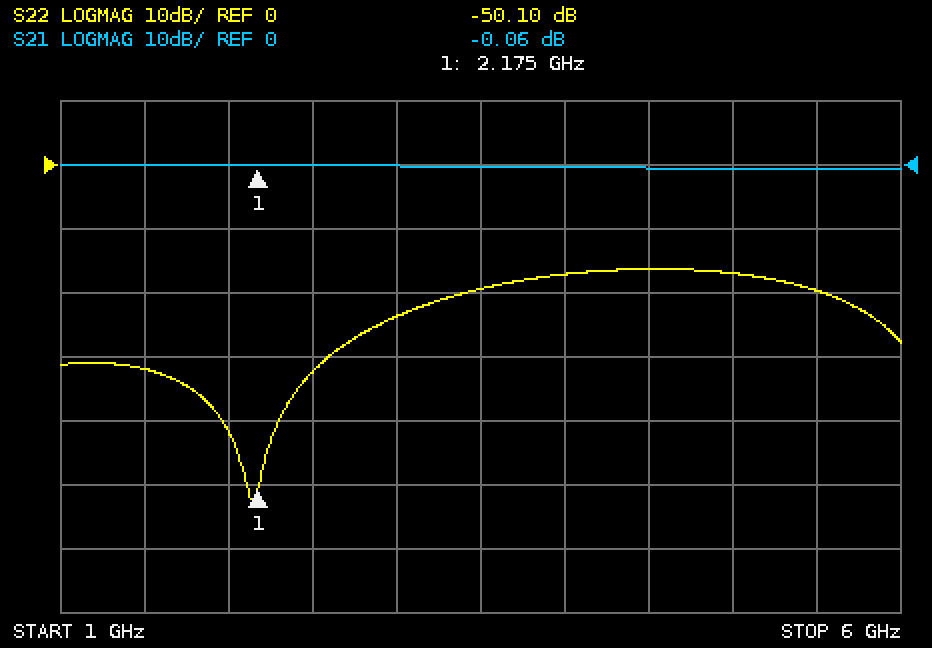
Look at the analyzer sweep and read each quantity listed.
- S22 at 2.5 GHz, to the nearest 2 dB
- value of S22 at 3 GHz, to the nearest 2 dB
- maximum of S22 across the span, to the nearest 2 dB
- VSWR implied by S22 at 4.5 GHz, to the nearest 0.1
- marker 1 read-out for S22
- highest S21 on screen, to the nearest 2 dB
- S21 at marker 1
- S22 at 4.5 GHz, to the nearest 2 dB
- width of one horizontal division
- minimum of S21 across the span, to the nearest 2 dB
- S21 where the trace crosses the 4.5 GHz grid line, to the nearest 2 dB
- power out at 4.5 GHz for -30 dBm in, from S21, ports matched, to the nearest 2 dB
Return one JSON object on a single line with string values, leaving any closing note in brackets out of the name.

{"S22 at 2.5 GHz, to the nearest 2 dB": "-32 dB", "value of S22 at 3 GHz, to the nearest 2 dB": "-24 dB", "maximum of S22 across the span, to the nearest 2 dB": "-16 dB", "VSWR implied by S22 at 4.5 GHz, to the nearest 0.1": "1.4", "marker 1 read-out for S22": "-50.10 dB", "highest S21 on screen, to the nearest 2 dB": "0 dB", "S21 at marker 1": "-0.06 dB", "S22 at 4.5 GHz, to the nearest 2 dB": "-16 dB", "width of one horizontal division": "500 MHz", "minimum of S21 across the span, to the nearest 2 dB": "0 dB", "S21 where the trace crosses the 4.5 GHz grid line, to the nearest 2 dB": "0 dB", "power out at 4.5 GHz for -30 dBm in, from S21, ports matched, to the nearest 2 dB": "-30 dBm"}
